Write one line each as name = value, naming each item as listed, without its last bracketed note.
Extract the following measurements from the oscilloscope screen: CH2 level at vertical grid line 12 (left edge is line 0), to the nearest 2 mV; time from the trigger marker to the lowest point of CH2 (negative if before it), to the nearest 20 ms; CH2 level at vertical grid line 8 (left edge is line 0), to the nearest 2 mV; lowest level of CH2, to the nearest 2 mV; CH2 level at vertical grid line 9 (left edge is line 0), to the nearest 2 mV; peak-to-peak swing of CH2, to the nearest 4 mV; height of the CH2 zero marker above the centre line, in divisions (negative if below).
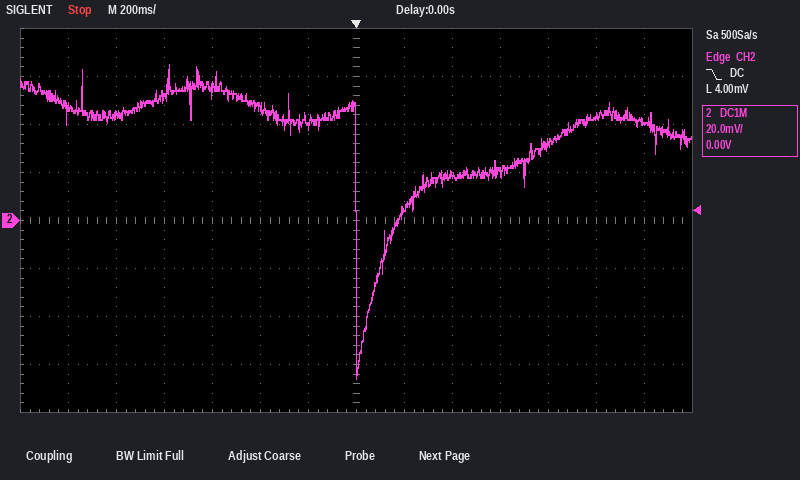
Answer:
CH2 level at vertical grid line 12 (left edge is line 0), to the nearest 2 mV = 44 mV
time from the trigger marker to the lowest point of CH2 (negative if before it), to the nearest 20 ms = 0 ms
CH2 level at vertical grid line 8 (left edge is line 0), to the nearest 2 mV = 4 mV
lowest level of CH2, to the nearest 2 mV = -66 mV
CH2 level at vertical grid line 9 (left edge is line 0), to the nearest 2 mV = 20 mV
peak-to-peak swing of CH2, to the nearest 4 mV = 132 mV
height of the CH2 zero marker above the centre line, in divisions = 0.0 div
